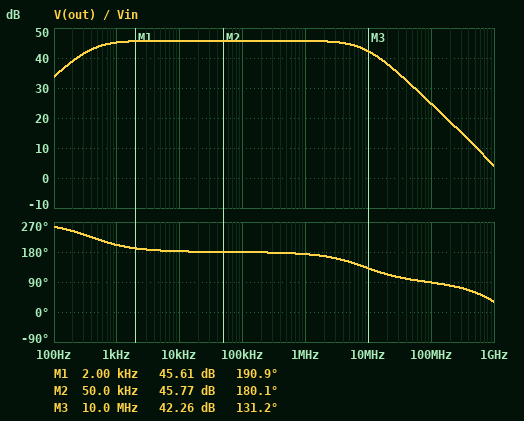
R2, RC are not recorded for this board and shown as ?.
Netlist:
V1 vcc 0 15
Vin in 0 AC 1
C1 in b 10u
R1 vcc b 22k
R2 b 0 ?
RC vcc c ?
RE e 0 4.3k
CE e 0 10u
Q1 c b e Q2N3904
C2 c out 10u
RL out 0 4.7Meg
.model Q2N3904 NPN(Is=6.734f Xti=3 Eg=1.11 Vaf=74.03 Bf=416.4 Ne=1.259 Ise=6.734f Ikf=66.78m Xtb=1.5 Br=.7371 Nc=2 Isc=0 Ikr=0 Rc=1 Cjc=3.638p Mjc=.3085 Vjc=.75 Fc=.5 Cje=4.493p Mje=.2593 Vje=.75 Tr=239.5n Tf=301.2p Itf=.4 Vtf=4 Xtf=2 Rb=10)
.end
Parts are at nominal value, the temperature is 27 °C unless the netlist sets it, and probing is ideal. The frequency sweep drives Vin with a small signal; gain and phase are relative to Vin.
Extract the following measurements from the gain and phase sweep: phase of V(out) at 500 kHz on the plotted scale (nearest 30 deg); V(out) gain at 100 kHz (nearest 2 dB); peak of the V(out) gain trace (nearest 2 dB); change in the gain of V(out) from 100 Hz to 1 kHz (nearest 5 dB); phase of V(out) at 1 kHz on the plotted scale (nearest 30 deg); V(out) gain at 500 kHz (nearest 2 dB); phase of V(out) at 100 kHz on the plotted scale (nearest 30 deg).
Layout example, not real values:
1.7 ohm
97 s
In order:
180 deg
46 dB
46 dB
10 dB
210 deg
46 dB
180 deg
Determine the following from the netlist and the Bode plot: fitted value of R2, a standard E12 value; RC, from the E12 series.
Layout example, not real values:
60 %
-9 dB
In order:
6.8 kΩ
8.2 kΩ
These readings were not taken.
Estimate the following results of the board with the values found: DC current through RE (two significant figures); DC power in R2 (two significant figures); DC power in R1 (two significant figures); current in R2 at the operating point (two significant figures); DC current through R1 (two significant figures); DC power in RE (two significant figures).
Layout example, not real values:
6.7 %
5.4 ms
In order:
670 µA
1.8 mW
6.0 mW
520 µA
520 µA
1.9 mW
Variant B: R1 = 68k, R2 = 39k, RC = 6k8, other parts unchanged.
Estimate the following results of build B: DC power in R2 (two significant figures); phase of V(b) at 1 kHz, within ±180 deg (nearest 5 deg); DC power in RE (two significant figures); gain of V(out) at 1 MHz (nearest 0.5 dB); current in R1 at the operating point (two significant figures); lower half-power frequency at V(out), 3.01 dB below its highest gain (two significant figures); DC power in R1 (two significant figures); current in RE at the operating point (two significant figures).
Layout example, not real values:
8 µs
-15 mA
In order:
710 µW
0 deg
4.9 mW
48.0 dB
140 µA
600 Hz
1.4 mW
1.1 mA
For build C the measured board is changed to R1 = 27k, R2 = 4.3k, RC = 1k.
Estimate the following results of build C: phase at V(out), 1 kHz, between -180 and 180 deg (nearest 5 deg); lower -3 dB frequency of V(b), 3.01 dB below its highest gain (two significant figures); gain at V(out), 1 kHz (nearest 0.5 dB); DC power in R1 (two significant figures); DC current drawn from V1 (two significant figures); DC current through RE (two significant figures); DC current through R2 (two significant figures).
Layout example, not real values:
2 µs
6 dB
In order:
-170 deg
4.3 Hz
22.0 dB
6.2 mW
810 µA
330 µA
480 µA
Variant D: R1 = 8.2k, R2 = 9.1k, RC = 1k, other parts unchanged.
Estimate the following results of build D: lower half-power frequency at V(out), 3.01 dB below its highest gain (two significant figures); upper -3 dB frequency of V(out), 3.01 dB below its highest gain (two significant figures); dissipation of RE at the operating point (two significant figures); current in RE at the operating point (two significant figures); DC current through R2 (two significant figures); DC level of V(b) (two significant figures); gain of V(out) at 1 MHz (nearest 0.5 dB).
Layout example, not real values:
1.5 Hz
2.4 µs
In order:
990 Hz
51 MHz
12 mW
1.7 mA
860 µA
7.8 V
35.5 dB
